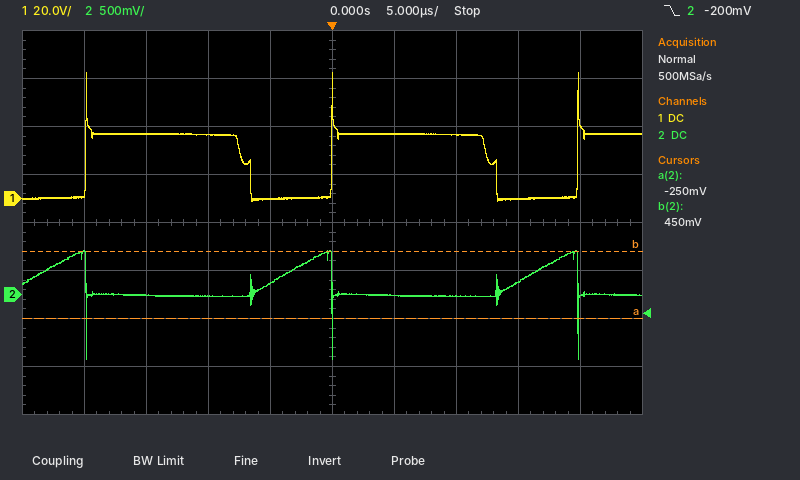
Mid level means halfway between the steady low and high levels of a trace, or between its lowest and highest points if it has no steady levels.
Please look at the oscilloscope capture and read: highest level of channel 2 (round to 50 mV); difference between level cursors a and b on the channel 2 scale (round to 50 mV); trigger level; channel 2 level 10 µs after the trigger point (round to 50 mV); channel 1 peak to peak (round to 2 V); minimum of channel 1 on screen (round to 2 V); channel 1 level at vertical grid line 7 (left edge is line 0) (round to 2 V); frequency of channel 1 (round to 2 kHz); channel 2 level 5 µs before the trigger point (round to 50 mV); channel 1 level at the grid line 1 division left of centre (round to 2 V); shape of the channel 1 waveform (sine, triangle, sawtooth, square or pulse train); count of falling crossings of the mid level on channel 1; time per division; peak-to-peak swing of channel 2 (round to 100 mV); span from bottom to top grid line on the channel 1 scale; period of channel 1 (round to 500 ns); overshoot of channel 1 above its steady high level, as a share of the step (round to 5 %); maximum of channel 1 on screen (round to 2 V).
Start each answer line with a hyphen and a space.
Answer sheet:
- 450 mV
- 700 mV
- -200 mV
- 0 mV
- 54 V
- -2 V
- 26 V
- 50 kHz
- 100 mV
- 0 V
- pulse train
- 2
- 5 µs
- 1.10 V
- 160 V
- 20.0 µs
- 95 %
- 52 V
